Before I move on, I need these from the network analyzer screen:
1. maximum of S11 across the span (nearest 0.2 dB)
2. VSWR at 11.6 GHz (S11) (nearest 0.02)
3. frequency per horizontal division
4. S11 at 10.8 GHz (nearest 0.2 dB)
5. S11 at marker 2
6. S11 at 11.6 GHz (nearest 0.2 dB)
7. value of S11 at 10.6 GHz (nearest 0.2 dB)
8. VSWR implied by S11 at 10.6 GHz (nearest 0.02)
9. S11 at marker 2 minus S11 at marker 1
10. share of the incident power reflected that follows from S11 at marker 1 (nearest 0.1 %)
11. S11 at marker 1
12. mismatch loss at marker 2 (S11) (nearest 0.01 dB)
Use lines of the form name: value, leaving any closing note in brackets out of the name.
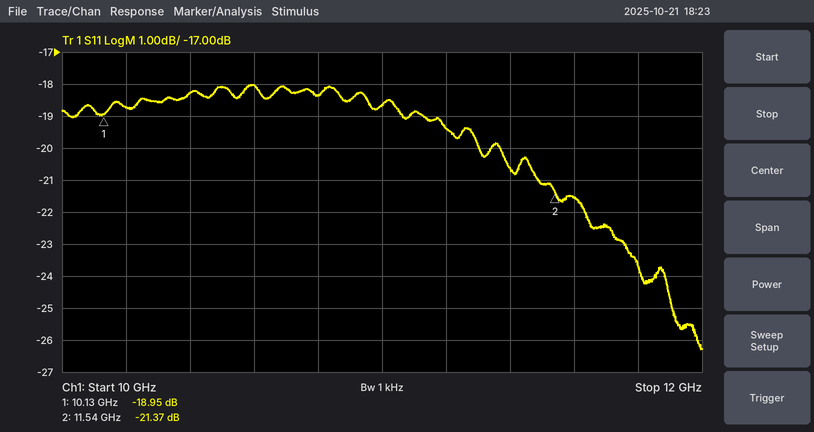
maximum of S11 across the span: -18.0 dB
VSWR at 11.6 GHz (S11): 1.18
frequency per horizontal division: 200 MHz
S11 at 10.8 GHz: -18.4 dB
S11 at marker 2: -21.37 dB
S11 at 11.6 GHz: -21.6 dB
value of S11 at 10.6 GHz: -18.0 dB
VSWR implied by S11 at 10.6 GHz: 1.28
S11 at marker 2 minus S11 at marker 1: -2.42 dB
share of the incident power reflected that follows from S11 at marker 1: 1.3 %
S11 at marker 1: -18.95 dB
mismatch loss at marker 2 (S11): 0.03 dB
